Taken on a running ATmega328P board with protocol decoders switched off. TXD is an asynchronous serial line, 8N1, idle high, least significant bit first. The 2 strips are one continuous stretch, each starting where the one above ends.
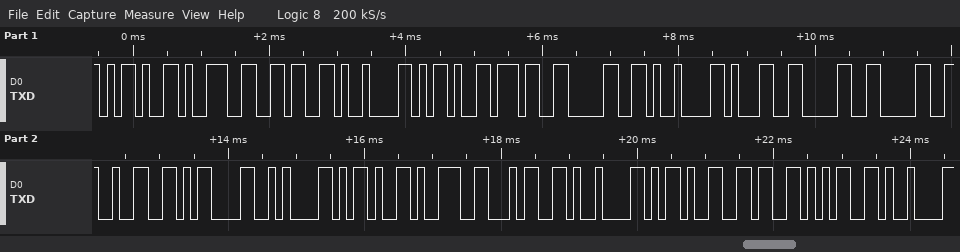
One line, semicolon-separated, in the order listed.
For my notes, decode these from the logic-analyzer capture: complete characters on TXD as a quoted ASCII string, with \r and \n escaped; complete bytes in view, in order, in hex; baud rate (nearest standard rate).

"-96\t-70\t1002\r\n-94\t-65\t"; 2D 39 36 09 2D 37 30 09 31 30 30 32 0D 0A 2D 39 34 09 2D 36 35 09; 9600 baud
